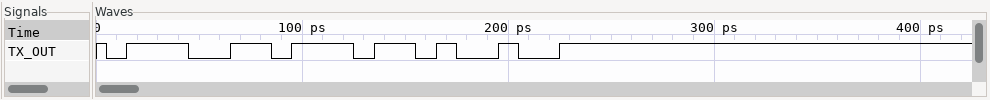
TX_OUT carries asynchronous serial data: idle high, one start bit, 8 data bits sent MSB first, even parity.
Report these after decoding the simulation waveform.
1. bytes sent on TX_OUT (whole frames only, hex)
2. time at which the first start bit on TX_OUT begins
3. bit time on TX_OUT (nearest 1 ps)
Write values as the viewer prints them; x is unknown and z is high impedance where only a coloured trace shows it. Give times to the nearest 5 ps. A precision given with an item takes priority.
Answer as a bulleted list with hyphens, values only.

- E6, D2
- 5 ps
- 10 ps
